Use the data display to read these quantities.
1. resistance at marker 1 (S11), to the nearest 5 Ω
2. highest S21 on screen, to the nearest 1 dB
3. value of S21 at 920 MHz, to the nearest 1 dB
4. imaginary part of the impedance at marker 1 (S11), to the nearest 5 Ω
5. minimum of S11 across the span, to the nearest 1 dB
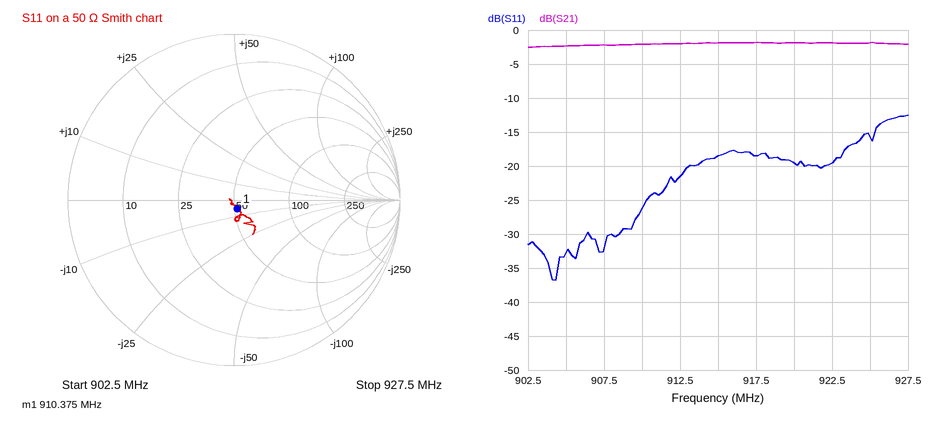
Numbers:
50 Ω
-2 dB
-2 dB
-5 Ω
-37 dB
